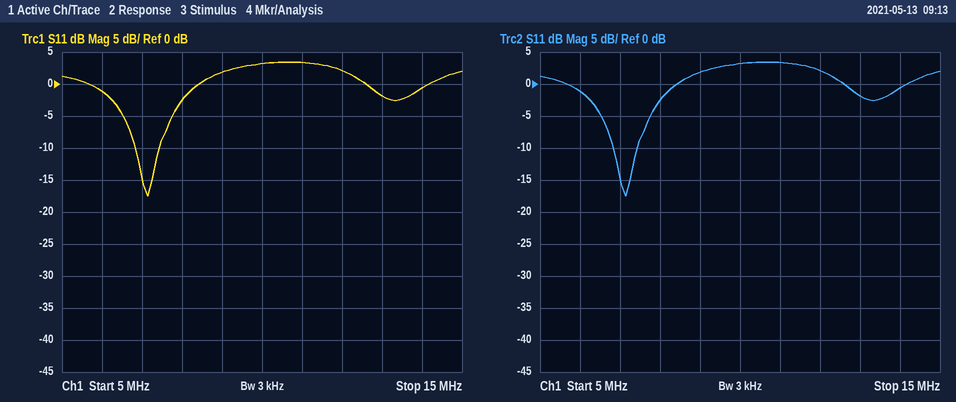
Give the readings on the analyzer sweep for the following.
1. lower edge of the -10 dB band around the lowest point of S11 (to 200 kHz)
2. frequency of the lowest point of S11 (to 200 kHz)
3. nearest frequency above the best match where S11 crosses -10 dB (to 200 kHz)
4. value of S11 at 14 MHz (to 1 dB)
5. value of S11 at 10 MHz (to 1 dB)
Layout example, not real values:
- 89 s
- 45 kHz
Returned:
- 6.8 MHz
- 7.2 MHz
- 7.4 MHz
- -1 dB
- 3 dB
